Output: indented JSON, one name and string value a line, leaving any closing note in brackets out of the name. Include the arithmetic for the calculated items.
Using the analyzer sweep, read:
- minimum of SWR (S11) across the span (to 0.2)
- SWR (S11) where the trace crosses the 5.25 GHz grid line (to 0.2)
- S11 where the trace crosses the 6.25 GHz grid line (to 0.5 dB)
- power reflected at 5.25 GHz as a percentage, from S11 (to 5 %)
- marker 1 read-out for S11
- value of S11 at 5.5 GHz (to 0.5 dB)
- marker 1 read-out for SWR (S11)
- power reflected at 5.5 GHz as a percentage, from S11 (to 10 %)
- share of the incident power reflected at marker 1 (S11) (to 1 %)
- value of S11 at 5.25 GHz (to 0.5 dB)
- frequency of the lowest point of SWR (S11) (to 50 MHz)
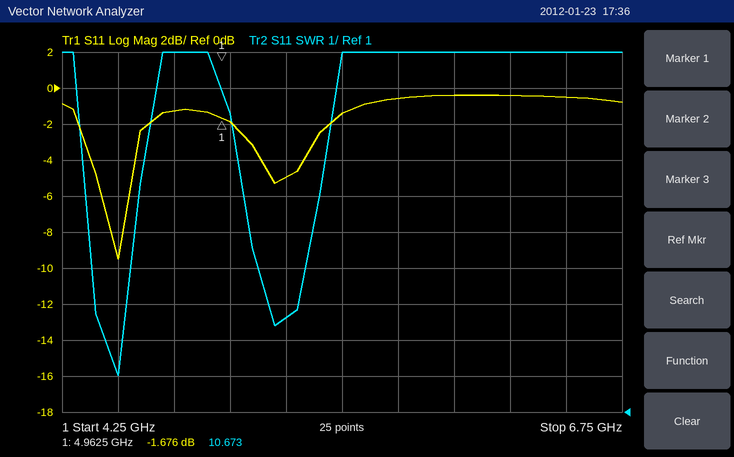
{
  "minimum of SWR (S11) across the span": "2.0",
  "SWR (S11) where the trace crosses the 5.25 GHz grid line": "3.6",
  "S11 where the trace crosses the 6.25 GHz grid line": "-0.5 dB",
  "power reflected at 5.25 GHz as a percentage, from S11": "10^(-5/10) ≈ 31.6 %, so 30 % to the nearest 5 %",
  "marker 1 read-out for S11": "-1.676 dB",
  "value of S11 at 5.5 GHz": "-1.5 dB",
  "marker 1 read-out for SWR": "10.673",
  "power reflected at 5.5 GHz as a percentage, from S11": "10^(-1.5/10) ≈ 70.8 %, so 70 % to the nearest 10 %",
  "share of the incident power reflected at marker 1 (S11)": "10^(-1.676/10) ≈ 68 %",
  "value of S11 at 5.25 GHz": "-5.0 dB",
  "frequency of the lowest point of SWR (S11)": "4.50 GHz"
}
